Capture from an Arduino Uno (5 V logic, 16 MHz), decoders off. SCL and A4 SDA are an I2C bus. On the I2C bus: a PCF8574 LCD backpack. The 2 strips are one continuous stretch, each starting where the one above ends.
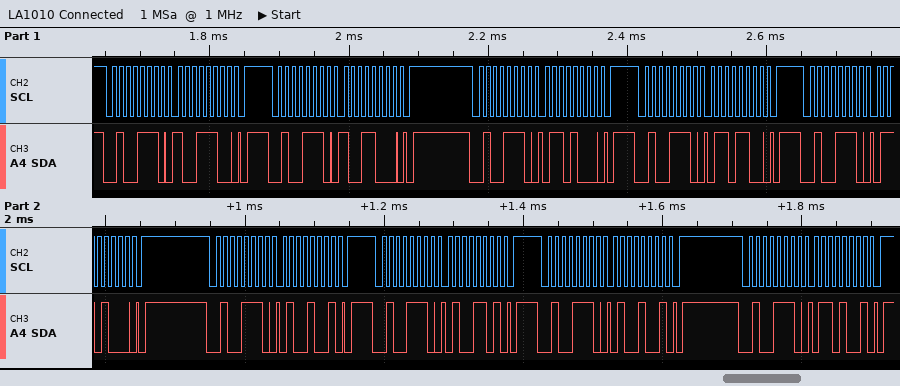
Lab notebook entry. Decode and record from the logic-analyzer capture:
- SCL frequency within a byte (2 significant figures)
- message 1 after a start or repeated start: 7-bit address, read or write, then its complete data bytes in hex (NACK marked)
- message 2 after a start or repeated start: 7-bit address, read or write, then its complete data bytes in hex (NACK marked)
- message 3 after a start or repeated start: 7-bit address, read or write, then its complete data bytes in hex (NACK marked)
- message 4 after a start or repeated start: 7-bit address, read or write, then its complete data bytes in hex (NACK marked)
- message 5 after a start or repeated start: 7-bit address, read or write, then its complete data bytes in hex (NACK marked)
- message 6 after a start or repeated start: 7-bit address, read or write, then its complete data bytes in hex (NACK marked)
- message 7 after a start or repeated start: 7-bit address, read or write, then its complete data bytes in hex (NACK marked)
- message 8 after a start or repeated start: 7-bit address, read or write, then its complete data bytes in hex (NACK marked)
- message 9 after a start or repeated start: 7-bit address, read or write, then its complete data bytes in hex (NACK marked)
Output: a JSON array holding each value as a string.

["100 kHz", "0x27 write: 9C", "0x27 write: 98", "0x27 write: 68", "0x27 write: 6C", "0x27 write: 68", "0x27 write: 49", "0x27 write: 4D", "0x27 write: 49", "0x27 write: 69"]
